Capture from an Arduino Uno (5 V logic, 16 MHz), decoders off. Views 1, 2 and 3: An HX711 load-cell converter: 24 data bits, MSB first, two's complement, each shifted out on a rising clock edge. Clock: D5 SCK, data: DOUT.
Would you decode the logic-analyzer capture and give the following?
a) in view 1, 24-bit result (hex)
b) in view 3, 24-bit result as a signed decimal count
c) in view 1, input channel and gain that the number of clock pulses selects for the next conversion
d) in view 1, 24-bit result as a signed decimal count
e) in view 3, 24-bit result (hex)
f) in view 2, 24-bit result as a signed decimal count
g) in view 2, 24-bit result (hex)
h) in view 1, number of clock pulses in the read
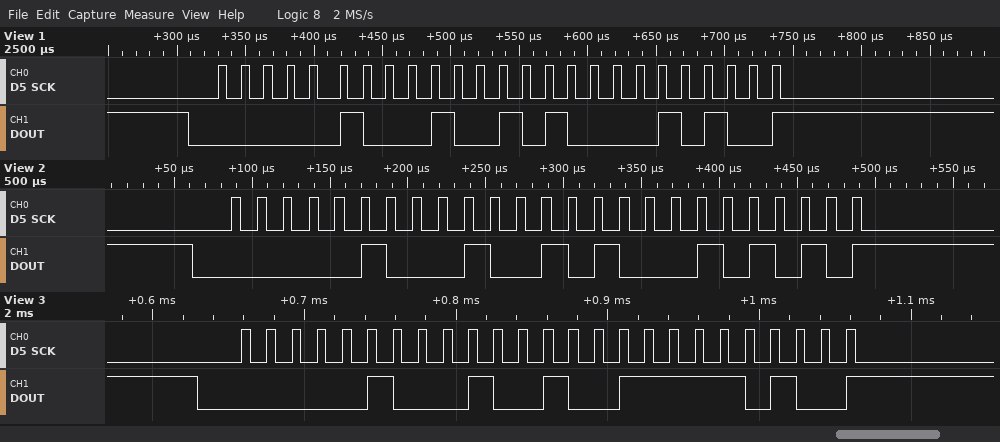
0x044A14
281076
channel A, gain 128
281108
0x0449F4
281130
0x044A2A
25
